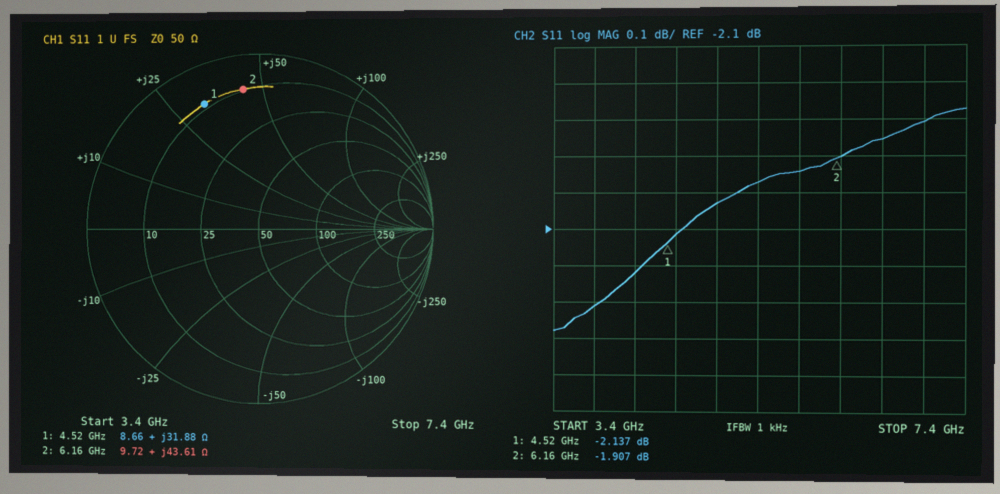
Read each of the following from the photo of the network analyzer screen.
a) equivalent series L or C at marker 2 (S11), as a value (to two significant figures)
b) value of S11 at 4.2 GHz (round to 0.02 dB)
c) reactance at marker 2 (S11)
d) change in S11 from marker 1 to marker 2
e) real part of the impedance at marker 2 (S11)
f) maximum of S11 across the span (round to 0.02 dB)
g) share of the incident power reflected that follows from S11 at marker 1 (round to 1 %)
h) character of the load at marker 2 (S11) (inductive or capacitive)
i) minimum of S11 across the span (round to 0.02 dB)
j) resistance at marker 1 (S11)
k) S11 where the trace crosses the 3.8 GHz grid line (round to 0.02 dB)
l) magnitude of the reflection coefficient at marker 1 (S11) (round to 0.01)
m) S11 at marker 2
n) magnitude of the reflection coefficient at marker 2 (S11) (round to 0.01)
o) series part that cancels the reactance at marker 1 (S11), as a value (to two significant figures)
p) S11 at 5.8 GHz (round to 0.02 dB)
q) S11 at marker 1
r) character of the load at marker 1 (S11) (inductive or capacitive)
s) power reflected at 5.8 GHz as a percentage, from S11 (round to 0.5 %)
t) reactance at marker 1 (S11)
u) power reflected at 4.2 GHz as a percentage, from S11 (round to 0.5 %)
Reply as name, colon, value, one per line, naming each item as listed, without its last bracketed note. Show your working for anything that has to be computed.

equivalent series L or C at marker 2 (S11), as a value: L = 43.61 Ω/(2π × 6.16 GHz) ≈ 1.1 nH
value of S11 at 4.2 GHz: -2.22 dB
reactance at marker 2: +43.61 Ω
change in S11 from marker 1 to marker 2: -1.907 − (-2.137) = 0.230 dB
real part of the impedance at marker 2: 9.72 Ω
maximum of S11 across the span: -1.78 dB
share of the incident power reflected that follows from S11 at marker 1: 10^(-2.137/10) ≈ 61 %
character of the load at marker 2 (S11): inductive
minimum of S11 across the span: -2.38 dB
resistance at marker 1: 8.66 Ω
S11 where the trace crosses the 3.8 GHz grid line: -2.32 dB
magnitude of the reflection coefficient at marker 1 (S11): 0.78
S11 at marker 2: -1.907 dB
magnitude of the reflection coefficient at marker 2 (S11): 0.80
series part that cancels the reactance at marker 1 (S11), as a value: C = 1/(2π × 4.52 GHz × 31.88 Ω) ≈ 1.1 pF
S11 at 5.8 GHz: -1.94 dB
S11 at marker 1: -2.137 dB
character of the load at marker 1 (S11): inductive
power reflected at 5.8 GHz as a percentage, from S11: 10^(-1.94/10) ≈ 64.0 %
reactance at marker 1: +31.88 Ω
power reflected at 4.2 GHz as a percentage, from S11: 10^(-2.22/10) ≈ 60.0 %
